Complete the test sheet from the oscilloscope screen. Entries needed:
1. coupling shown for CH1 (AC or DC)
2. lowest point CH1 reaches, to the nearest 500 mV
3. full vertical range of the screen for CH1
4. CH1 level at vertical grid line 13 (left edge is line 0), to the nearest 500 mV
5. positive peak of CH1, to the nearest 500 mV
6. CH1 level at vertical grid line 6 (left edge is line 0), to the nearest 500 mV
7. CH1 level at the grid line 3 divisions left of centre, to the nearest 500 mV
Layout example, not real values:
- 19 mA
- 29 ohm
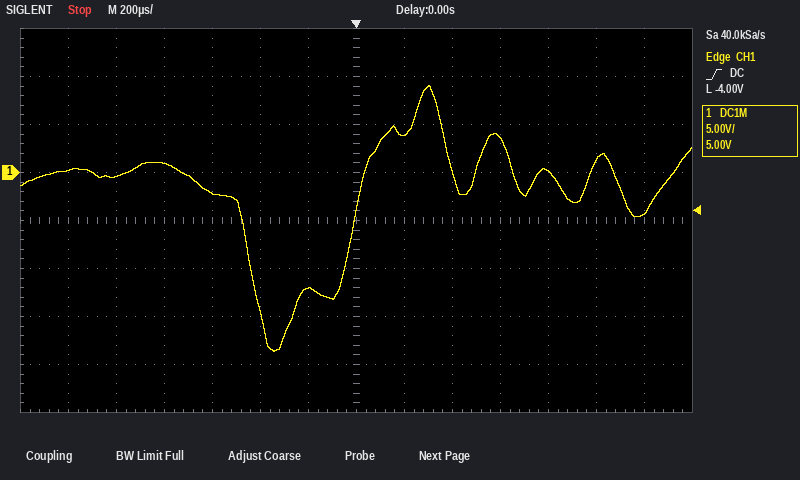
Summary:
- DC
- -18.5 V
- 40 V
- -4.5 V
- 9.0 V
- -12.0 V
- -2.0 V
